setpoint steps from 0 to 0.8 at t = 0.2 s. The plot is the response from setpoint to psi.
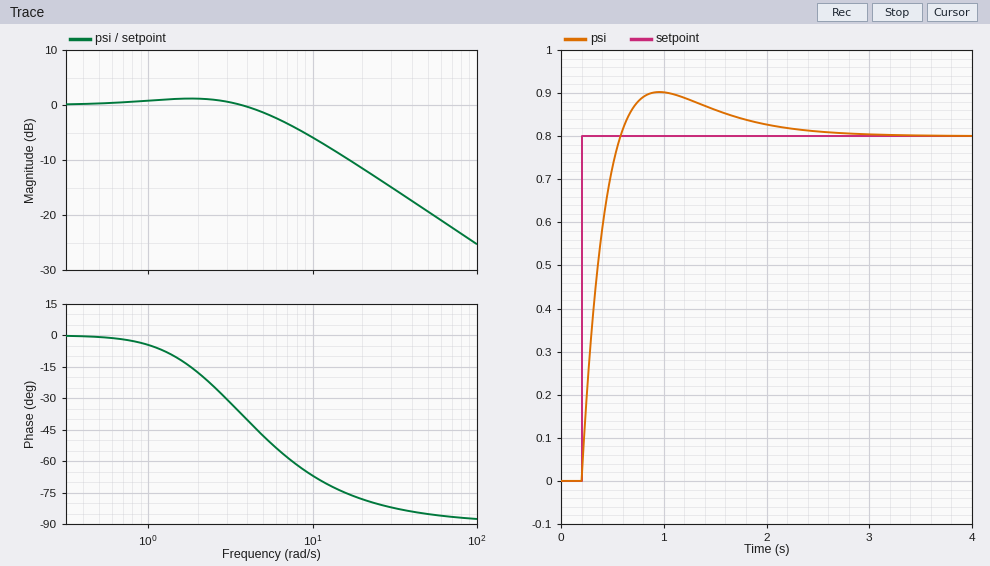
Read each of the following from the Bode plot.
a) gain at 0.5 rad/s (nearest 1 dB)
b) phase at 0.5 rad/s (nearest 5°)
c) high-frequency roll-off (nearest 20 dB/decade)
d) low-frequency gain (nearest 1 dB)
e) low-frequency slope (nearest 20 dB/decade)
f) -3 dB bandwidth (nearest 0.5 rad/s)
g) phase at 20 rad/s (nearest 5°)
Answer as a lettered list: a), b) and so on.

a) 0 dB
b) 0°
c) -20 dB/decade
d) 0 dB
e) 0 dB/decade
f) 6.5 rad/s
g) -80°
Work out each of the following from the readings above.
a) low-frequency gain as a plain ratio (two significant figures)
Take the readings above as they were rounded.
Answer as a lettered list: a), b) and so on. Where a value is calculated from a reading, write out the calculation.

a) 10^(0 / 20) = 1.0
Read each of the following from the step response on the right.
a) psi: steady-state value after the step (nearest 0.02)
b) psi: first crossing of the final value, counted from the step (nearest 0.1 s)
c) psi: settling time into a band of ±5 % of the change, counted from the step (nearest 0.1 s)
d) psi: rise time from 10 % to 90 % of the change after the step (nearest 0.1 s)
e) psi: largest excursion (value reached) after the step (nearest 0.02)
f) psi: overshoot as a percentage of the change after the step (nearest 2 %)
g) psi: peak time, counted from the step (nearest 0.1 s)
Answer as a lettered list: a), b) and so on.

a) 0.80
b) 0.4 s
c) 1.6 s
d) 0.3 s
e) 0.90
f) 12 %
g) 0.8 s
